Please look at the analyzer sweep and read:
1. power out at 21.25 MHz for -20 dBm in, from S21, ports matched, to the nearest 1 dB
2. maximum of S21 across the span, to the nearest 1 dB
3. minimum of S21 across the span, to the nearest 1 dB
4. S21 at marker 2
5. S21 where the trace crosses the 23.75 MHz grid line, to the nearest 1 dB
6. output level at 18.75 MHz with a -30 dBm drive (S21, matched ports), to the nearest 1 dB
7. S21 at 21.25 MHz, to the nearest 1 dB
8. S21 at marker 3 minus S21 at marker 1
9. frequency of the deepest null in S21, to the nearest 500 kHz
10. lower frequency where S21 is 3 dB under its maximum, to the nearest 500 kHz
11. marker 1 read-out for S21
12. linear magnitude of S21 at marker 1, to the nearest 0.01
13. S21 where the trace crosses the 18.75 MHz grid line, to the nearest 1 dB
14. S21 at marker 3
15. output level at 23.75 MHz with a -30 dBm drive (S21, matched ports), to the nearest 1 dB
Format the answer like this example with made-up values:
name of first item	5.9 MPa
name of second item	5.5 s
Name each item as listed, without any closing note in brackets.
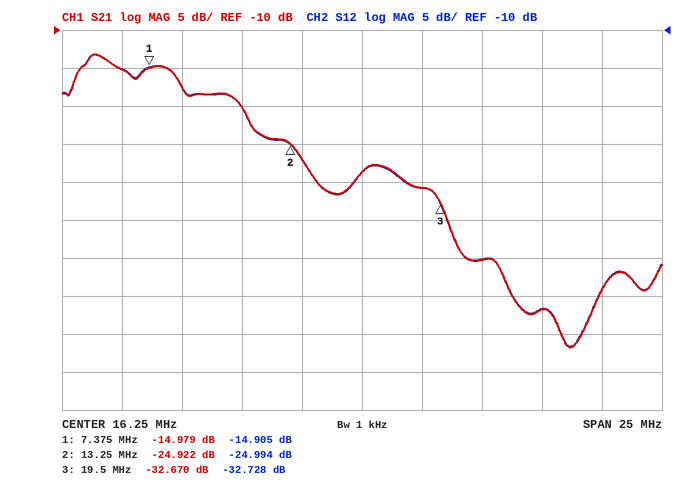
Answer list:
power out at 21.25 MHz for -20 dBm in, from S21, ports matched, to the nearest 1 dB	-60 dBm
maximum of S21 across the span, to the nearest 1 dB	-13 dB
minimum of S21 across the span, to the nearest 1 dB	-52 dB
S21 at marker 2	-24.922 dB
S21 where the trace crosses the 23.75 MHz grid line, to the nearest 1 dB	-47 dB
output level at 18.75 MHz with a -30 dBm drive (S21, matched ports), to the nearest 1 dB	-61 dBm
S21 at 21.25 MHz, to the nearest 1 dB	-40 dB
S21 at marker 3 minus S21 at marker 1	-17.691 dB
frequency of the deepest null in S21, to the nearest 500 kHz	25.0 MHz
lower frequency where S21 is 3 dB under its maximum, to the nearest 500 kHz	4.5 MHz
marker 1 read-out for S21	-14.979 dB
linear magnitude of S21 at marker 1, to the nearest 0.01	0.18
S21 where the trace crosses the 18.75 MHz grid line, to the nearest 1 dB	-31 dB
S21 at marker 3	-32.670 dB
output level at 23.75 MHz with a -30 dBm drive (S21, matched ports), to the nearest 1 dB	-77 dBm
